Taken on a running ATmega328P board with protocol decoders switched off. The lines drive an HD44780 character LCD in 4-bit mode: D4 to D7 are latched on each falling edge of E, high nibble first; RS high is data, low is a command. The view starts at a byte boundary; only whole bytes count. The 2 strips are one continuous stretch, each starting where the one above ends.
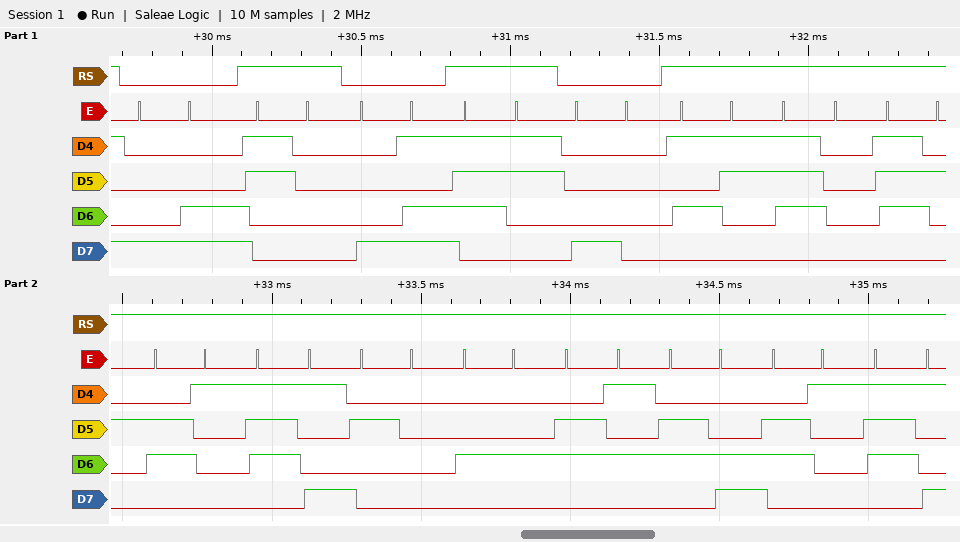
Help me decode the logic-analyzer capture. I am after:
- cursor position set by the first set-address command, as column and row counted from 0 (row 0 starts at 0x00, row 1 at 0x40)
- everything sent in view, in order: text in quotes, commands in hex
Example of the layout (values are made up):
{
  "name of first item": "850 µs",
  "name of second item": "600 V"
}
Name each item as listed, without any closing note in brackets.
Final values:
{
  "cursor position set by the first set-address command, as column and row counted from 0": "column 12, row 0",
  "everything sent in view, in order: text in quotes, commands in hex": "0x8C \"0\" 0x8D \"s\" 0x80 \"Spray Delay\""
}
